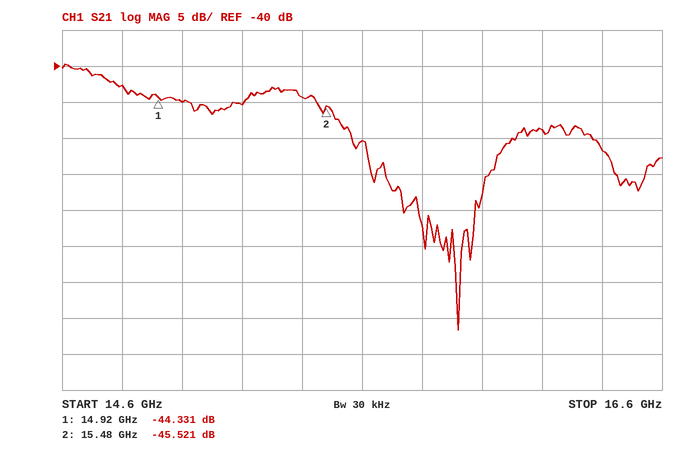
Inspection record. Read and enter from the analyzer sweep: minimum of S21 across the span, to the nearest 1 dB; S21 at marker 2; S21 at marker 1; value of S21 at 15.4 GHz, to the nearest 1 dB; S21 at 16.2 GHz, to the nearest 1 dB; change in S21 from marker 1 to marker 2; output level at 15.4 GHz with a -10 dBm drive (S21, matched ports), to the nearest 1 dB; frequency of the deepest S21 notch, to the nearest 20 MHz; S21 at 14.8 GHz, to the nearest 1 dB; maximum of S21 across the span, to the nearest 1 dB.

-77 dB
-45.521 dB
-44.331 dB
-44 dB
-49 dB
-1.190 dB
-54 dBm
15.92 GHz
-43 dB
-40 dB
